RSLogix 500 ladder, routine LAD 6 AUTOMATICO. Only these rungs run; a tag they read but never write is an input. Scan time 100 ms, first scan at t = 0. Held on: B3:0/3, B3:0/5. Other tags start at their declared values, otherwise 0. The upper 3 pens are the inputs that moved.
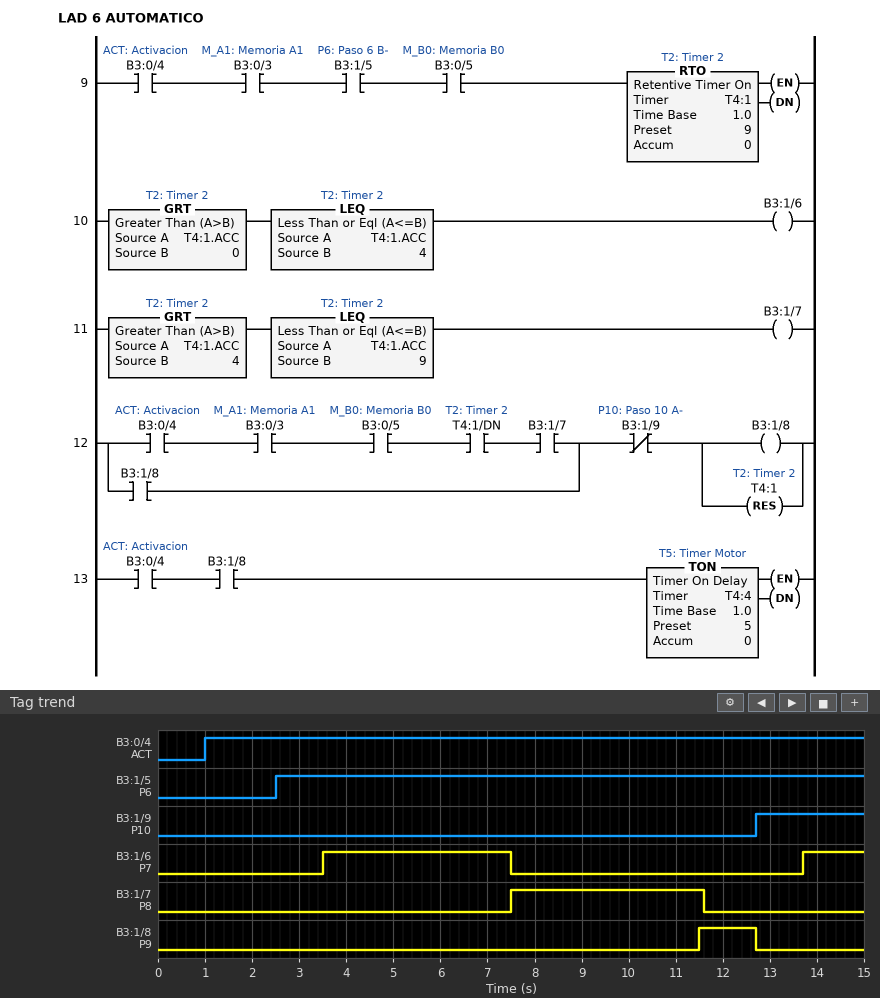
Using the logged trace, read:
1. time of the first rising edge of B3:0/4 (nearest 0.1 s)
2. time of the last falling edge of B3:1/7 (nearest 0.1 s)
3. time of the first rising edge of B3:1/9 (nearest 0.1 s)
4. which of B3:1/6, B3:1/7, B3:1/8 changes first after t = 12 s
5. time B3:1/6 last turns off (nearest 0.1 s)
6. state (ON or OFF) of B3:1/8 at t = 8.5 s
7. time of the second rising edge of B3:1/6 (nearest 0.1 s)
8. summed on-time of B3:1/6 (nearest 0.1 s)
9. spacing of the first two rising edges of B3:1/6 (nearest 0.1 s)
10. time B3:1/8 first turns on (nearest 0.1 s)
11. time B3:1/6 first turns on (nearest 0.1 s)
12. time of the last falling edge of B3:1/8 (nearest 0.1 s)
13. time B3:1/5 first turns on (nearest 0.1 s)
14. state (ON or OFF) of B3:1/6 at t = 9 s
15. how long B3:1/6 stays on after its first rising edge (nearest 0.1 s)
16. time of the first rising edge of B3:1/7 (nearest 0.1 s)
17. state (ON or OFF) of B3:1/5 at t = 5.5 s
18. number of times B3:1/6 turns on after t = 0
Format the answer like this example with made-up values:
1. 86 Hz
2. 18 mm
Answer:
1. 1.0 s
2. 11.6 s
3. 12.7 s
4. B3:1/8
5. 7.5 s
6. OFF
7. 13.7 s
8. 5.3 s
9. 10.2 s
10. 11.5 s
11. 3.5 s
12. 12.7 s
13. 2.5 s
14. OFF
15. 4.0 s
16. 7.5 s
17. ON
18. 2
